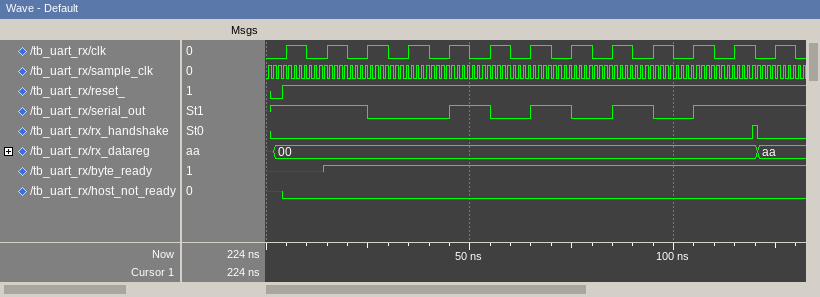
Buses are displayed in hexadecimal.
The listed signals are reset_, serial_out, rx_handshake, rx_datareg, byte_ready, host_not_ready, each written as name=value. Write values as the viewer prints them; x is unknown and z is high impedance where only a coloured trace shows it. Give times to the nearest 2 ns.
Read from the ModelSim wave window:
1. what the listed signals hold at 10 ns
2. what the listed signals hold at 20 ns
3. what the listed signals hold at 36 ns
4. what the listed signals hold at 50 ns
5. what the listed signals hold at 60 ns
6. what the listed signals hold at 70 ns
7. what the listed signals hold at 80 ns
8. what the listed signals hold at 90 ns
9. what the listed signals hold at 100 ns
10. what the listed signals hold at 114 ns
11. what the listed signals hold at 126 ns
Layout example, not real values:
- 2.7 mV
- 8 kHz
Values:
- reset_=1, serial_out=1, rx_handshake=0, rx_datareg=00, byte_ready=x, host_not_ready=0
- reset_=1, serial_out=1, rx_handshake=0, rx_datareg=00, byte_ready=1, host_not_ready=0
- reset_=1, serial_out=0, rx_handshake=0, rx_datareg=00, byte_ready=1, host_not_ready=0
- reset_=1, serial_out=1, rx_handshake=0, rx_datareg=00, byte_ready=1, host_not_ready=0
- reset_=1, serial_out=0, rx_handshake=0, rx_datareg=00, byte_ready=1, host_not_ready=0
- reset_=1, serial_out=1, rx_handshake=0, rx_datareg=00, byte_ready=1, host_not_ready=0
- reset_=1, serial_out=0, rx_handshake=0, rx_datareg=00, byte_ready=1, host_not_ready=0
- reset_=1, serial_out=1, rx_handshake=0, rx_datareg=00, byte_ready=1, host_not_ready=0
- reset_=1, serial_out=0, rx_handshake=0, rx_datareg=00, byte_ready=1, host_not_ready=0
- reset_=1, serial_out=1, rx_handshake=0, rx_datareg=00, byte_ready=1, host_not_ready=0
- reset_=1, serial_out=1, rx_handshake=0, rx_datareg=aa, byte_ready=1, host_not_ready=0
